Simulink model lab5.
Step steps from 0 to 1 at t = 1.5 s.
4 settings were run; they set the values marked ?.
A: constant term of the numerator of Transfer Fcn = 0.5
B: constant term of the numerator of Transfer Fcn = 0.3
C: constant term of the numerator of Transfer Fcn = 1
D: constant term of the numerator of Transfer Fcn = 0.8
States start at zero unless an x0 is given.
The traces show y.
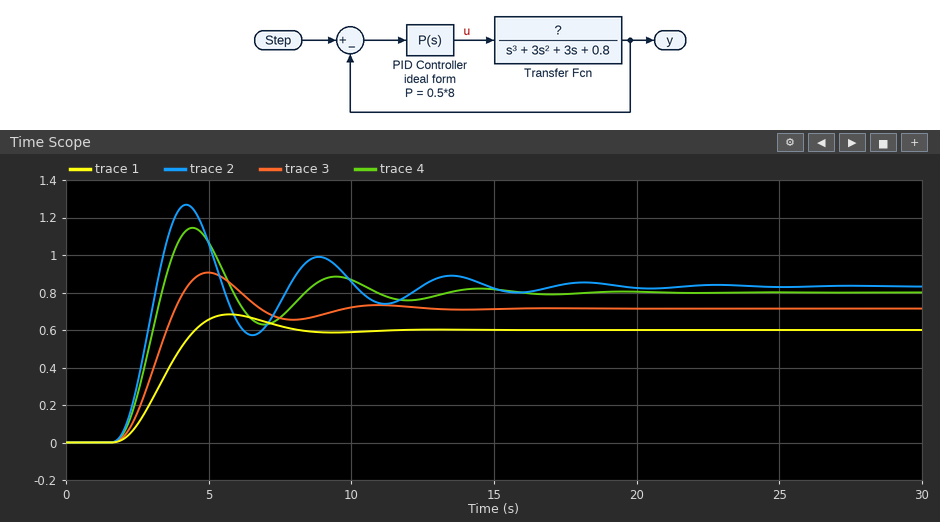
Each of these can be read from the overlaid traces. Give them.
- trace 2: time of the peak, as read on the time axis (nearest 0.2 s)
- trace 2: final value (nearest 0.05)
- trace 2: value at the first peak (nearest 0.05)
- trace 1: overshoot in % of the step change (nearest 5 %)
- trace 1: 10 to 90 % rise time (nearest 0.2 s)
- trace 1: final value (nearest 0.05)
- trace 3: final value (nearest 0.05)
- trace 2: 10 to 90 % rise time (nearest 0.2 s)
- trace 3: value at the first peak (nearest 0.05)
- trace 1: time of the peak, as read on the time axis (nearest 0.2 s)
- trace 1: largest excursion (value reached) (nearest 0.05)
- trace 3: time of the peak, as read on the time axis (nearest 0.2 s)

4.2 s
0.85
1.25
15 %
1.8 s
0.60
0.70
1.0 s
0.90
5.8 s
0.70
5.0 s
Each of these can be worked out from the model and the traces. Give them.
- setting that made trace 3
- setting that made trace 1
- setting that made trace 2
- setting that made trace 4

A
B
C
D
